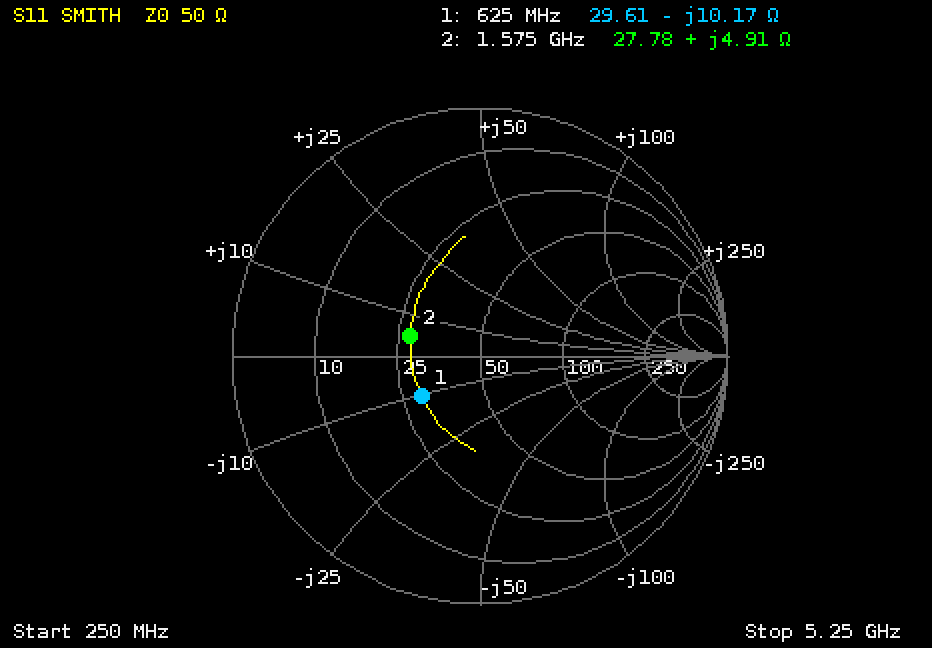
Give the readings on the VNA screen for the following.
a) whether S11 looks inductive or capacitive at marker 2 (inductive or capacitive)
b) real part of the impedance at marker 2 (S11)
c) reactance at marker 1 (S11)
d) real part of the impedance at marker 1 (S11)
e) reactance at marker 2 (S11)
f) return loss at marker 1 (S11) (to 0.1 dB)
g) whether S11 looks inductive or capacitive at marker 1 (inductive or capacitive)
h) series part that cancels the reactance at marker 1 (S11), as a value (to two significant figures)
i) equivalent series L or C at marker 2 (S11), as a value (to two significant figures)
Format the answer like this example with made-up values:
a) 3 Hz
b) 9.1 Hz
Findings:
a) inductive
b) 27.78 Ω
c) -10.17 Ω
d) 29.61 Ω
e) +4.91 Ω
f) 10.9 dB
g) capacitive
h) 2.6 nH
i) 500 pH
